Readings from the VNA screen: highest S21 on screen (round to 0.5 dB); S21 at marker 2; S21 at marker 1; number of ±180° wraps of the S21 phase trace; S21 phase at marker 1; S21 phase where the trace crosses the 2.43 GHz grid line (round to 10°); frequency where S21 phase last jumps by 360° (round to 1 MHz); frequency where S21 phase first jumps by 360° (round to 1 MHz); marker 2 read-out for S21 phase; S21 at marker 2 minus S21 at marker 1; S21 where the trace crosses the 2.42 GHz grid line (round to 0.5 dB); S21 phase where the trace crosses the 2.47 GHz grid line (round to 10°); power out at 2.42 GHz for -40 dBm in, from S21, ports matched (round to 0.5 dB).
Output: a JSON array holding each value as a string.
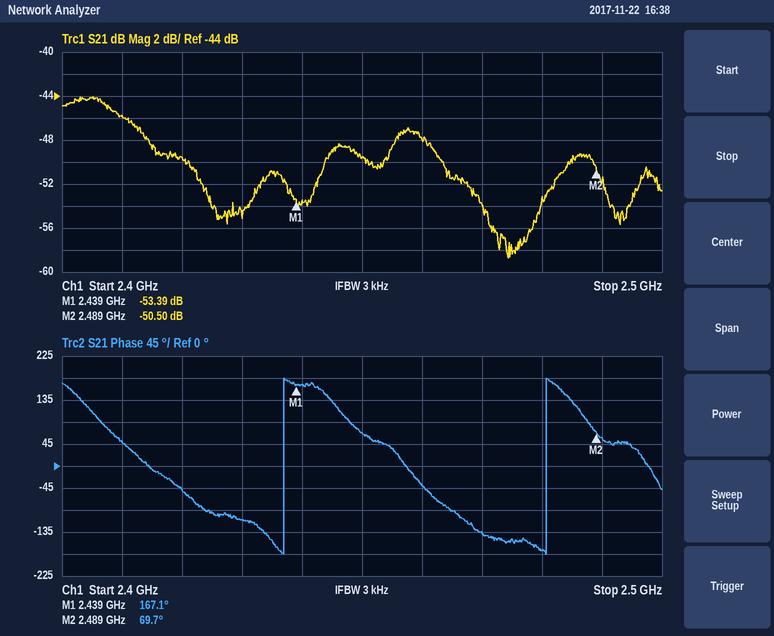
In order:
["-44.0 dB", "-50.50 dB", "-53.39 dB", "2", "167.1°", "-110°", "2.481 GHz", "2.437 GHz", "69.7°", "2.89 dB", "-49.5 dB", "-140°", "-89.5 dBm"]
